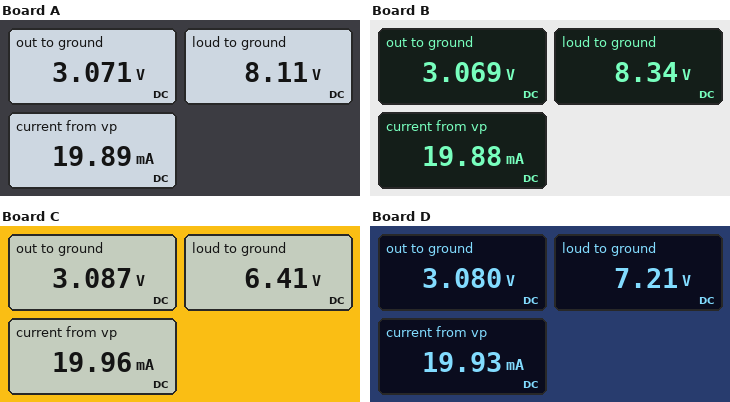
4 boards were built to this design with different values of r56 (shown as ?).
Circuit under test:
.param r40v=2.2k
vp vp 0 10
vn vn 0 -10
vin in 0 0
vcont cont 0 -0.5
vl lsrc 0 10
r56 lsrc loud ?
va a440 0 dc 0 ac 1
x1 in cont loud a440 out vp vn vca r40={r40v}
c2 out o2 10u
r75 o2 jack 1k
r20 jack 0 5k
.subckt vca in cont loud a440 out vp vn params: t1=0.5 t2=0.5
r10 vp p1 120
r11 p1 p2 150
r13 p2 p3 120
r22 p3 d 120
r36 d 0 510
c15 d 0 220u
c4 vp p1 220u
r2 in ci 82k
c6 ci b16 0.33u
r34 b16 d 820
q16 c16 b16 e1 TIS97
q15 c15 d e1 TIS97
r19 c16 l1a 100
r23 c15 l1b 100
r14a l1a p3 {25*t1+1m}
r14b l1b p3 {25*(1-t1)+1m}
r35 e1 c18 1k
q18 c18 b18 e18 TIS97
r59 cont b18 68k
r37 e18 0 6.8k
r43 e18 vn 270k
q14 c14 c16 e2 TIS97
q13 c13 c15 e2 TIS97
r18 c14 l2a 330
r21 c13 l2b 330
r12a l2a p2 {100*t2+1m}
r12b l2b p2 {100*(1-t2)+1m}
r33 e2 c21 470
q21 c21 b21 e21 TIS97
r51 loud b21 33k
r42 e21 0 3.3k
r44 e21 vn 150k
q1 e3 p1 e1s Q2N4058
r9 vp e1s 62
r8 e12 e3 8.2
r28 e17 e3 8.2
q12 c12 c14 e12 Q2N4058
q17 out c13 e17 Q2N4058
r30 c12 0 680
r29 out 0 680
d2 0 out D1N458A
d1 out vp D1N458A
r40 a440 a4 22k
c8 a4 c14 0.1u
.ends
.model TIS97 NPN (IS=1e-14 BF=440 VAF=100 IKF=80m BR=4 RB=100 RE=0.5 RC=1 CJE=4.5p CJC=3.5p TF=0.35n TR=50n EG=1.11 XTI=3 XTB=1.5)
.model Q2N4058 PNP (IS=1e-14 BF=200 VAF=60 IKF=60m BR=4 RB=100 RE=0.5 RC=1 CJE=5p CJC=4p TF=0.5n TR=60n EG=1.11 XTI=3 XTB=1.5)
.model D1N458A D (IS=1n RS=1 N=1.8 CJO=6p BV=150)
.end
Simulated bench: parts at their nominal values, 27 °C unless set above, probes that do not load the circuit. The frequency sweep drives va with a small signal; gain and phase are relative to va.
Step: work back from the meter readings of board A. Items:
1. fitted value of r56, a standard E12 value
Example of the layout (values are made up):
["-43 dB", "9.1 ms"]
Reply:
["22 kΩ"]
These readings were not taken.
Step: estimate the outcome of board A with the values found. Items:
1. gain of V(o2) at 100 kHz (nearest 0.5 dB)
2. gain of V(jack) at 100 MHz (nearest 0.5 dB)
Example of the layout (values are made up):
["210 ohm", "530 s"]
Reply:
["-11.0 dB", "-55.5 dB"]
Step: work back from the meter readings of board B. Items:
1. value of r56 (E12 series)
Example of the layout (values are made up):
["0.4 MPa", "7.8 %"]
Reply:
["18 kΩ"]
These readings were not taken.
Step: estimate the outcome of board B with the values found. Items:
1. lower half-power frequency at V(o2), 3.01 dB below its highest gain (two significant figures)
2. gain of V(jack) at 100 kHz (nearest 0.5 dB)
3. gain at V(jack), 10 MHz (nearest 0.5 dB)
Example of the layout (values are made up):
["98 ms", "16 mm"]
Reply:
["71 Hz", "-12.5 dB", "-24.5 dB"]
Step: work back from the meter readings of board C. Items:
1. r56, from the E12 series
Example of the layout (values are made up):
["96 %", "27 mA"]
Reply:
["100 kΩ"]
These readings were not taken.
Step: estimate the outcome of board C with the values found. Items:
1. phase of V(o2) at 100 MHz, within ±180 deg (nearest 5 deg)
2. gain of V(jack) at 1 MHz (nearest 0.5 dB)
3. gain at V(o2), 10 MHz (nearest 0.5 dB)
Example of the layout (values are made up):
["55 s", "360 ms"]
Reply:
["-135 deg", "-13.0 dB", "-23.0 dB"]
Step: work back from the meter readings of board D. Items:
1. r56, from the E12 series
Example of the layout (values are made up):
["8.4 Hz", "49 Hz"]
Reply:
["47 kΩ"]
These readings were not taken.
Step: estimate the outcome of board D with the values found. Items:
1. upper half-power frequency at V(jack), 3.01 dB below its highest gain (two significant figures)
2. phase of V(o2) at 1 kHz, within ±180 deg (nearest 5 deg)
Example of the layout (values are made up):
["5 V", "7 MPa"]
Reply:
["2.6 MHz", "5 deg"]
